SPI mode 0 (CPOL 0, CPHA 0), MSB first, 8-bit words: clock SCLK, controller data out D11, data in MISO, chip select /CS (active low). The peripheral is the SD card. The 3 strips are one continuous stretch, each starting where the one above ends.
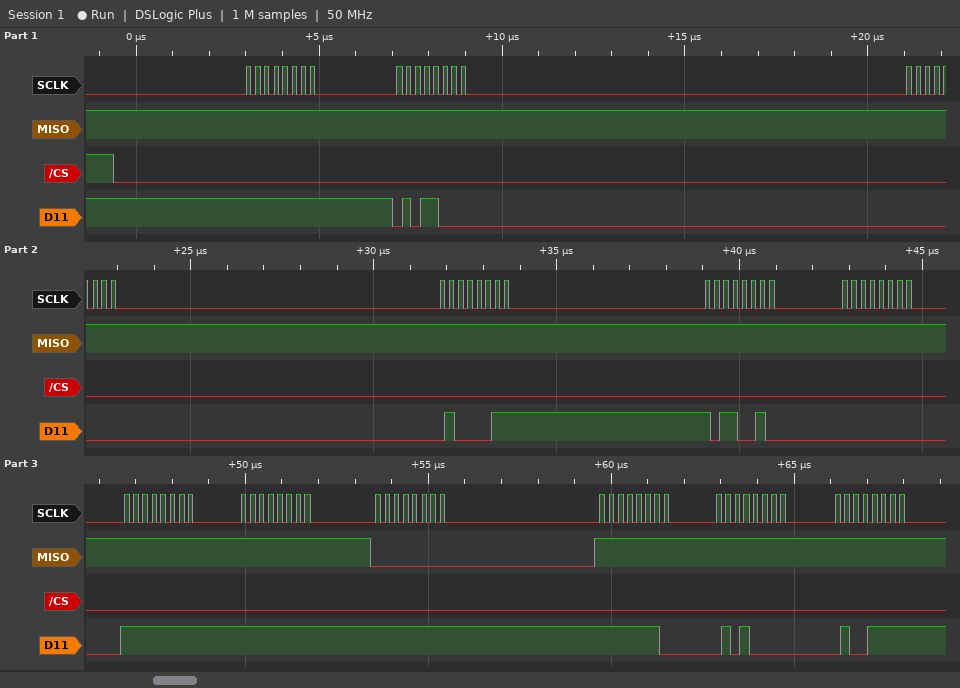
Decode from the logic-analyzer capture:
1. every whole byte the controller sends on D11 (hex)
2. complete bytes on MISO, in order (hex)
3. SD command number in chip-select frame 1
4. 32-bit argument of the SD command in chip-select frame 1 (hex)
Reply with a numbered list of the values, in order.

1. 0xFF 0x58 0x00 0x43 0xB2 0x00 0xFF 0xFF 0xFF 0xFE 0x50 0x4F
2. 0xFF 0xFF 0xFF 0xFF 0xFF 0xFF 0xFF 0xFF 0x00 0xFF 0xFF 0xFF
3. CMD24
4. 0x0043B200
